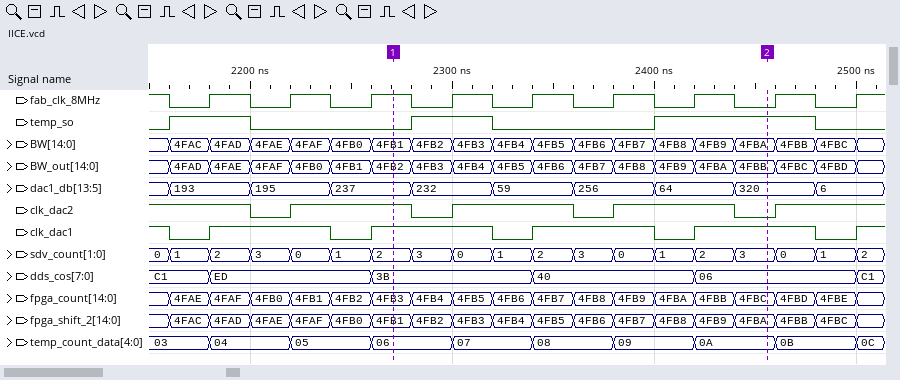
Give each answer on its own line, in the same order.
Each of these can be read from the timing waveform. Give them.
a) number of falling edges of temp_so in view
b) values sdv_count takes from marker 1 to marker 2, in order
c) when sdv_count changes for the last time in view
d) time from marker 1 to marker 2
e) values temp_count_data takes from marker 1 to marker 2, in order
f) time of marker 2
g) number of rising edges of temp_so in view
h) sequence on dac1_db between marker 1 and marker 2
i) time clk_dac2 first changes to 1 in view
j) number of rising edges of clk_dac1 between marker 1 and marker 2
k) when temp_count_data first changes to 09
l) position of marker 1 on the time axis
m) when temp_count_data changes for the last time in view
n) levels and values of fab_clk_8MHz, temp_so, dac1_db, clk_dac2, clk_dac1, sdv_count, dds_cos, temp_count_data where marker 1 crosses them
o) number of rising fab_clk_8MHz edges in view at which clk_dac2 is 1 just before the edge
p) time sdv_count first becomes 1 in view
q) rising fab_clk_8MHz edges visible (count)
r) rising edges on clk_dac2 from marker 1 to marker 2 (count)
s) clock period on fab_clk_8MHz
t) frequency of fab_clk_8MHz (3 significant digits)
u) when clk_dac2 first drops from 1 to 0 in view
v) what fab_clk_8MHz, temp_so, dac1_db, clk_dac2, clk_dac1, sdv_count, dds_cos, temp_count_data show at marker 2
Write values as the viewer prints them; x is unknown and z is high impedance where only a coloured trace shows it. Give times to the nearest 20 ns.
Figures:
3
2, 3, 0, 1, 2, 3, 0, 1, 2, 3
2500 ns
180 ns
06, 07, 08, 09, 0A
2460 ns
3
237, 232, 59, 256, 64, 320
2220 ns
2
2380 ns
2280 ns
2500 ns
fab_clk_8MHz=1, temp_so=0, dac1_db=237, clk_dac2=1, clk_dac1=1, sdv_count=2, dds_cos=3B, temp_count_data=06
5
2160 ns
9
2
40 ns
25.0 MHz
2200 ns
fab_clk_8MHz=0, temp_so=1, dac1_db=320, clk_dac2=0, clk_dac1=1, sdv_count=3, dds_cos=06, temp_count_data=0A
